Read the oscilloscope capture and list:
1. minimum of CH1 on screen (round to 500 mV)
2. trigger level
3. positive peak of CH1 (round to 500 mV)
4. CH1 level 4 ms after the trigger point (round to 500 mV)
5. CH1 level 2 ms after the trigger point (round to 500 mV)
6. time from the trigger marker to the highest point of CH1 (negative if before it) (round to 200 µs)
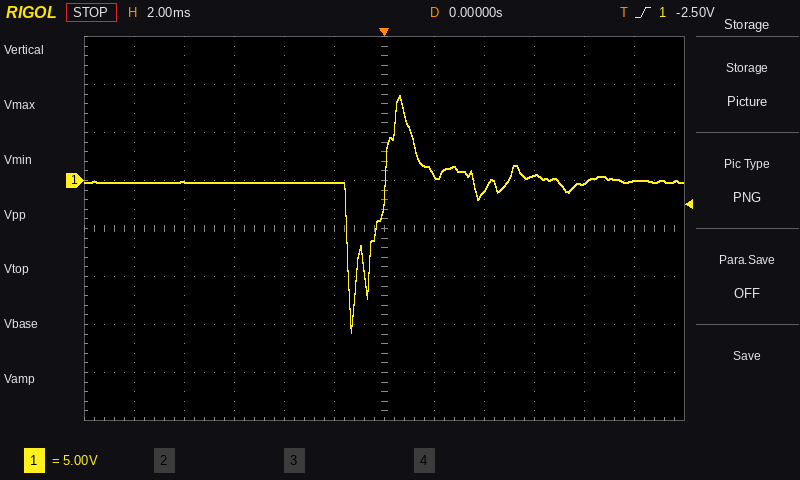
-16.0 V
-2.50 V
9.0 V
-1.0 V
500 mV
+600 µs
